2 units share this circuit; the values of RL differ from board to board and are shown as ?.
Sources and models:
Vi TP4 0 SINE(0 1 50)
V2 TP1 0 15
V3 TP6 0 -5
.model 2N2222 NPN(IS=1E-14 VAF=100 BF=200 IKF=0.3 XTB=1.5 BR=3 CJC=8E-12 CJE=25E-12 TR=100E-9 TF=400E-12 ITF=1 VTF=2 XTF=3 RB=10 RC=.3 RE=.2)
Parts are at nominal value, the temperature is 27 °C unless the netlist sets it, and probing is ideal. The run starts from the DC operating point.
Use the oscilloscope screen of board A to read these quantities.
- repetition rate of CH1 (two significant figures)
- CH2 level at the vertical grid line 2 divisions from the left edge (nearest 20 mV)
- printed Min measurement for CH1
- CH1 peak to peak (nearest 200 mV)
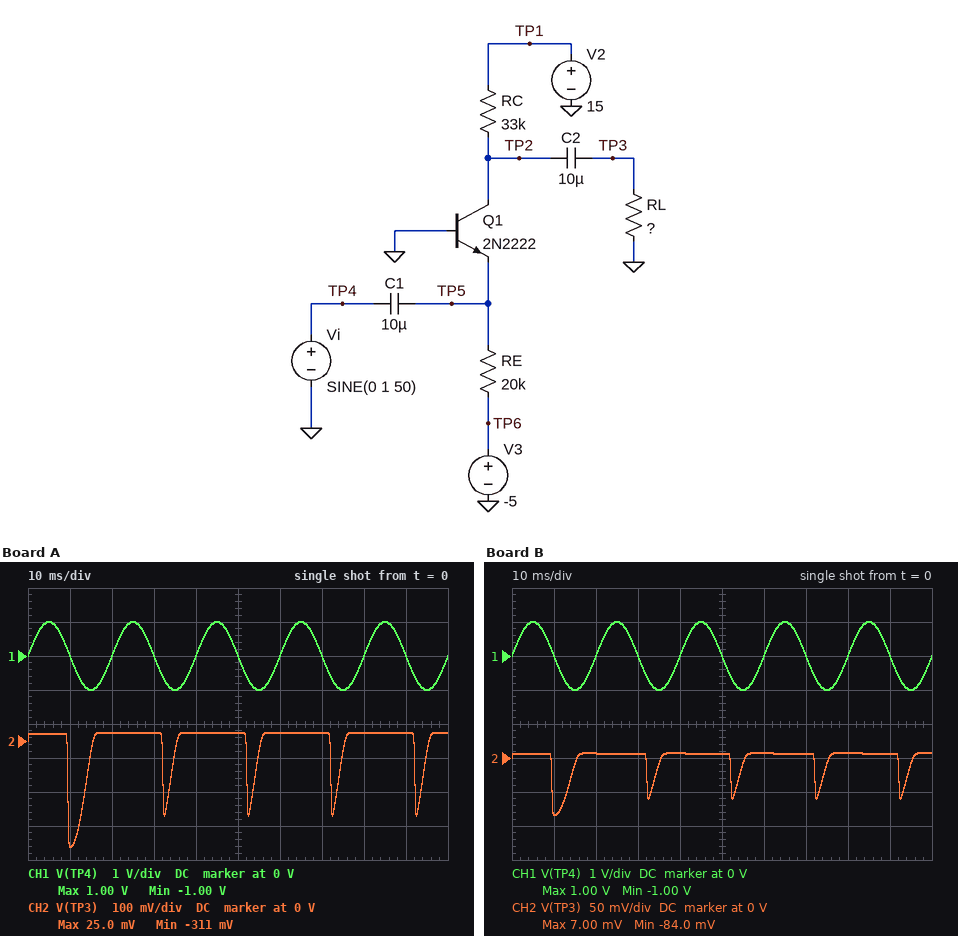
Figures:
50 Hz
20 mV
-1.00 V
2.0 V
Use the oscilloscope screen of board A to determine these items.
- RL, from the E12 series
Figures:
100 Ω
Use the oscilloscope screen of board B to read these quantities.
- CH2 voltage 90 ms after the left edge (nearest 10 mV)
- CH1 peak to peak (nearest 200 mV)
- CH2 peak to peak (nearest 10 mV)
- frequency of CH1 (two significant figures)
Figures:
10 mV
2.0 V
90 mV
50 Hz
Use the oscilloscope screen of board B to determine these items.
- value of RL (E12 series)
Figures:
27 Ω
